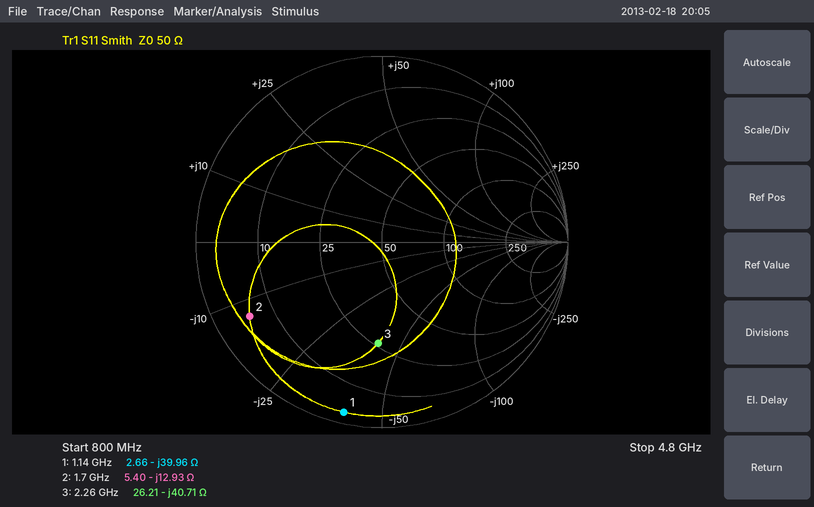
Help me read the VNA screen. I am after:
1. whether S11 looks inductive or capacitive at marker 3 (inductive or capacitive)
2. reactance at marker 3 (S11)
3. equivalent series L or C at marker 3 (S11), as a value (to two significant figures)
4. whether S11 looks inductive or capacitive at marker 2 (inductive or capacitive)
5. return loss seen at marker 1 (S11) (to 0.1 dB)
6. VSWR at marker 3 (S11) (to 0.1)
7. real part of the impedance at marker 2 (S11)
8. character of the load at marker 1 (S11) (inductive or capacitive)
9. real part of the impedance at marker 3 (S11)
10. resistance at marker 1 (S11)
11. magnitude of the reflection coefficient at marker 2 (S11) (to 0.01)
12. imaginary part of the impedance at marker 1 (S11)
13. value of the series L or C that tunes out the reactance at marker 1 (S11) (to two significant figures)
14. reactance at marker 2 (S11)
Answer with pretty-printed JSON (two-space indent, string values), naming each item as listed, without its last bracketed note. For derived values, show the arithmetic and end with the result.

{
  "whether S11 looks inductive or capacitive at marker 3": "capacitive",
  "reactance at marker 3": "-40.71 Ω",
  "equivalent series L or C at marker 3 (S11), as a value": "C = 1/(2π × 2.26 GHz × 40.71 Ω) ≈ 1.7 pF",
  "whether S11 looks inductive or capacitive at marker 2": "capacitive",
  "return loss seen at marker 1 (S11)": "0.6 dB",
  "VSWR at marker 3 (S11)": "3.4",
  "real part of the impedance at marker 2": "5.40 Ω",
  "character of the load at marker 1 (S11)": "capacitive",
  "real part of the impedance at marker 3": "26.21 Ω",
  "resistance at marker 1": "2.66 Ω",
  "magnitude of the reflection coefficient at marker 2 (S11)": "0.82",
  "imaginary part of the impedance at marker 1": "-39.96 Ω",
  "value of the series L or C that tunes out the reactance at marker 1 (S11)": "L = 39.96 Ω/(2π × 1.14 GHz) ≈ 5.6 nH",
  "reactance at marker 2": "-12.93 Ω"
}
